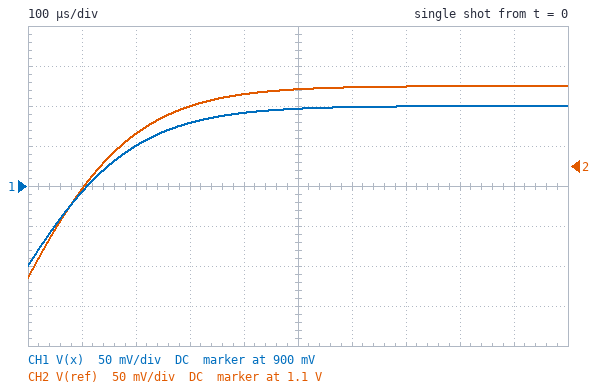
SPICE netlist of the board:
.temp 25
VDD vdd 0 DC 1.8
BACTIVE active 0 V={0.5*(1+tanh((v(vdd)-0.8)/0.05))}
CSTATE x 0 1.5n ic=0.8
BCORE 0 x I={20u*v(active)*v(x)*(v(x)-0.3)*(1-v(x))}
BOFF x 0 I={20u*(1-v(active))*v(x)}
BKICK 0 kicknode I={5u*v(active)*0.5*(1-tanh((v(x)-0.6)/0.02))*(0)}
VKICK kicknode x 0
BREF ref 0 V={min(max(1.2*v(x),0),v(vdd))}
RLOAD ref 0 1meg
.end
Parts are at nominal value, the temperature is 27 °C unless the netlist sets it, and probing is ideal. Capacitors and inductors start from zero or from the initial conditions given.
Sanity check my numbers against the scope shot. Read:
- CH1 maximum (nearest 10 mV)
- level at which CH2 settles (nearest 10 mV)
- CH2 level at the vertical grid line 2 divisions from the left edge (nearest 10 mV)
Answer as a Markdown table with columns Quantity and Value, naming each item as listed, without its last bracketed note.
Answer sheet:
| Quantity | Value |
|---|---|
| CH1 maximum | 1.00 V |
| level at which CH2 settles | 1.20 V |
| CH2 level at the vertical grid line 2 divisions from the left edge | 1.14 V |
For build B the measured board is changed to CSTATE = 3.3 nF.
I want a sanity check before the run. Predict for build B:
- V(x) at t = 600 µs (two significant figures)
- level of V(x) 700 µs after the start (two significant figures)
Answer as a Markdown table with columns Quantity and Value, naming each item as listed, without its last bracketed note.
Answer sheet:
| Quantity | Value |
|---|---|
| V(x) at t = 600 µs | 970 mV |
| level of V(x) 700 µs after the start | 980 mV |
